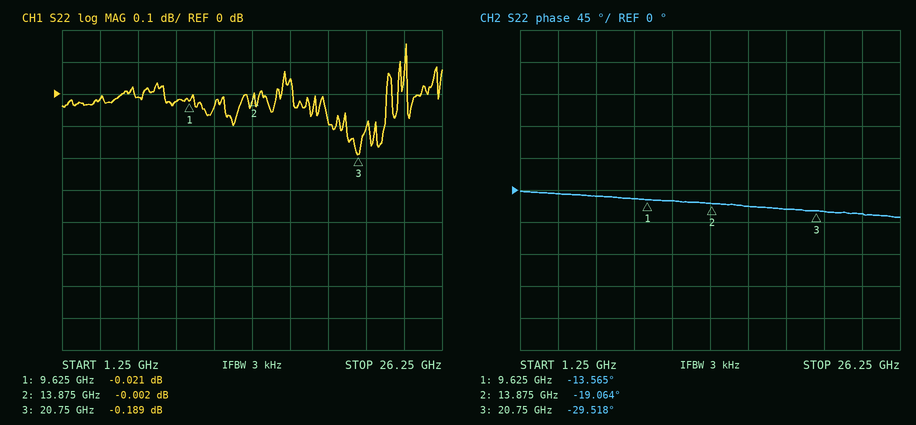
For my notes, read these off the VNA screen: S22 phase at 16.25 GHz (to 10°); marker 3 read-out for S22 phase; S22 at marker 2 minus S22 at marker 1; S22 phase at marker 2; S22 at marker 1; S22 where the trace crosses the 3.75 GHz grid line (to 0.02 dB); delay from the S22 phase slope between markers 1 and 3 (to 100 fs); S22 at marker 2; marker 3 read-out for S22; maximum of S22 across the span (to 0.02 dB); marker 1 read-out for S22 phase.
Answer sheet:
-20°
-29.518°
0.019 dB
-19.064°
-0.021 dB
-0.02 dB
4.0 ps
-0.002 dB
-0.189 dB
0.16 dB
-13.565°
